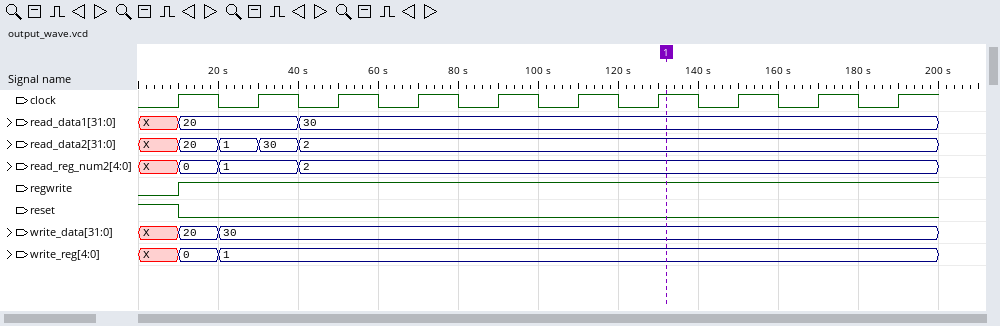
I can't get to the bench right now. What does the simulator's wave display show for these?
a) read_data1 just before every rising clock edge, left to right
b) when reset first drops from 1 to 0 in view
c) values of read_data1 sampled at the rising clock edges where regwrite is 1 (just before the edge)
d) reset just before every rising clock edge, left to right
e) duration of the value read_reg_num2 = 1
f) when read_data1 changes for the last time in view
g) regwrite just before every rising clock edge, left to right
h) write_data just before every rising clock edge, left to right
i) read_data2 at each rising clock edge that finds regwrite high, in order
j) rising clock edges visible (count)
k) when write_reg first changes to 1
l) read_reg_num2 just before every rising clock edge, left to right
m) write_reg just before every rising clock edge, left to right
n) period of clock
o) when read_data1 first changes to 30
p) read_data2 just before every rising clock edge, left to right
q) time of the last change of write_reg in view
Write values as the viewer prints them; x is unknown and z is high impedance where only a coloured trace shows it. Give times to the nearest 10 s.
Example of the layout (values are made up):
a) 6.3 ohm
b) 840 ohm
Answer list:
a) X, 20, 30, 30, 30, 30, 30, 30, 30, 30
b) 10 s
c) 20, 30, 30, 30, 30, 30, 30, 30, 30
d) 1 0 0 0 0 0 0 0 0 0
e) 20 s
f) 40 s
g) 0 1 1 1 1 1 1 1 1 1
h) X, 30, 30, 30, 30, 30, 30, 30, 30, 30
i) 1, 2, 2, 2, 2, 2, 2, 2, 2
j) 10
k) 20 s
l) X, 1, 2, 2, 2, 2, 2, 2, 2, 2
m) X, 1, 1, 1, 1, 1, 1, 1, 1, 1
n) 20 s
o) 40 s
p) X, 1, 2, 2, 2, 2, 2, 2, 2, 2
q) 20 s
